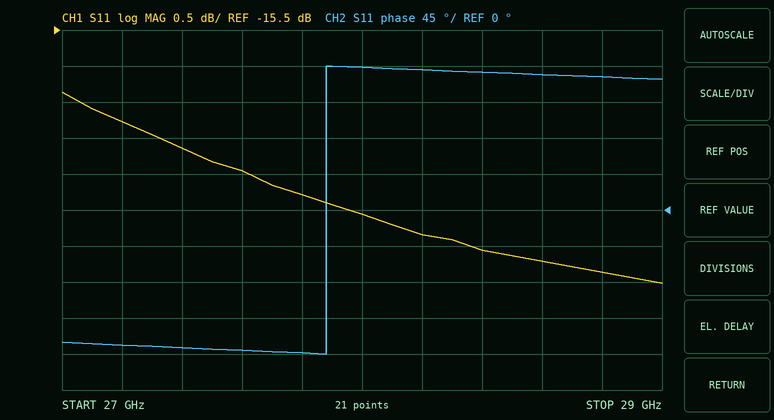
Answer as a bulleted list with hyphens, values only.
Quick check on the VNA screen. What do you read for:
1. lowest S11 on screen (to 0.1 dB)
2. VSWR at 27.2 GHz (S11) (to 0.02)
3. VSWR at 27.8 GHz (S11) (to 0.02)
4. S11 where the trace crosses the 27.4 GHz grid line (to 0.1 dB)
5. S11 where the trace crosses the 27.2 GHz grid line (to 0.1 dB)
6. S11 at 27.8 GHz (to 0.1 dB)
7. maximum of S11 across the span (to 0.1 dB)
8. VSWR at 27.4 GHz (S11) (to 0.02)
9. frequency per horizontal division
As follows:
- -19.0 dB
- 1.34
- 1.30
- -17.1 dB
- -16.8 dB
- -17.8 dB
- -16.4 dB
- 1.32
- 200 MHz
